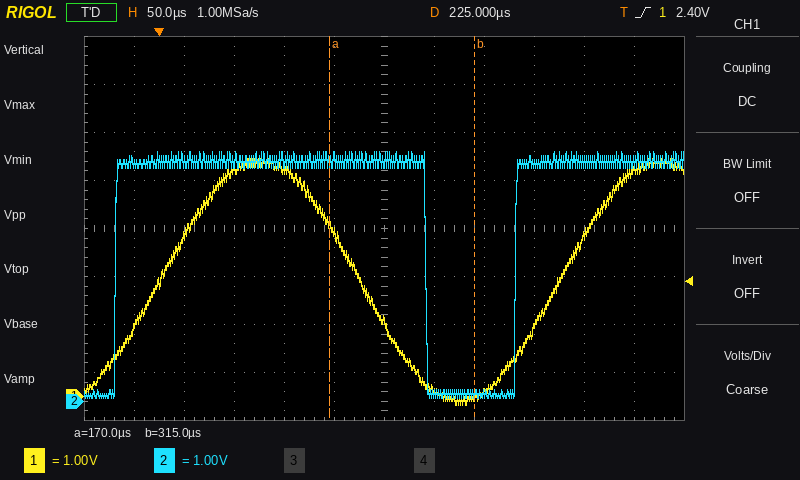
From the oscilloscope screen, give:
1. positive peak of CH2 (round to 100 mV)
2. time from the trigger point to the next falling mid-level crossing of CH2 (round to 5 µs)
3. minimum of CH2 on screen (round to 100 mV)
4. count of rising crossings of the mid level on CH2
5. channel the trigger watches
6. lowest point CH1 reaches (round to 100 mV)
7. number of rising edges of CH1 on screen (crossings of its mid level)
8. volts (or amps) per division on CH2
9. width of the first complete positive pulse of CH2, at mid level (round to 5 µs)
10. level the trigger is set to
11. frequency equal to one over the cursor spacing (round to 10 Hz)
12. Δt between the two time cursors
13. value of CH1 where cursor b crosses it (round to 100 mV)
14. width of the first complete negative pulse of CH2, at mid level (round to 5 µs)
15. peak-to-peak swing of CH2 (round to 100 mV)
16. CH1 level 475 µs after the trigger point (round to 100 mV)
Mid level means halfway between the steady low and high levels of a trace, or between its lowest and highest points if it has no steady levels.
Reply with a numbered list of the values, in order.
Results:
1. 5.2 V
2. 265 µs
3. 100 mV
4. 2
5. CH1
6. -200 mV
7. 2
8. 1 V
9. 310 µs
10. 2.40 V
11. 6.90 kHz
12. 145 µs
13. 0.0 V
14. 90 µs
15. 5.1 V
16. 4.7 V
